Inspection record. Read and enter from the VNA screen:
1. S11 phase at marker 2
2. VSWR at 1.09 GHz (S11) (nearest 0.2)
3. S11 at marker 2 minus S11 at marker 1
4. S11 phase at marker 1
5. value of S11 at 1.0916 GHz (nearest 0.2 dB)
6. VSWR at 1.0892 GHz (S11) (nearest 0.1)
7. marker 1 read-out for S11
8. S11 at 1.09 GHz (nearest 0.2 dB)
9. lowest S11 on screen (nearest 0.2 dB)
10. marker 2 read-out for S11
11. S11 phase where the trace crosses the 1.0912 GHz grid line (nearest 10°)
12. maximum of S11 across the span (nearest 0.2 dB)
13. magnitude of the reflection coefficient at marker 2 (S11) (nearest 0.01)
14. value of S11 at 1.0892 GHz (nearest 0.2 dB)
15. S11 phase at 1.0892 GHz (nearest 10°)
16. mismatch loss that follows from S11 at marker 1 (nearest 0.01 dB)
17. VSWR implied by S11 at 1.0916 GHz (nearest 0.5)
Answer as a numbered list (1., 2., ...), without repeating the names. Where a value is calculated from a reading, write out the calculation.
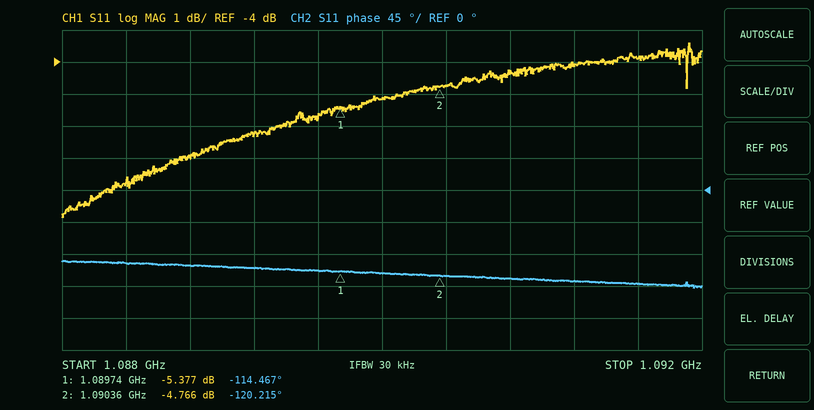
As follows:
1. -120.215°
2. |Γ| = 10^(-5.2/20) = 0.5495; VSWR = (1 + 0.5495)/(1 − 0.5495) ≈ 3.4
3. -4.766 − (-5.377) = 0.611 dB
4. -114.467°
5. -3.8 dB
6. |Γ| = 10^(-6.2/20) = 0.4898; VSWR = (1 + 0.4898)/(1 − 0.4898) ≈ 2.9
7. -5.377 dB
8. -5.2 dB
9. -8.8 dB
10. -4.766 dB
11. -130°
12. -3.4 dB
13. 10^(-4.766/20) ≈ 0.58
14. -6.2 dB
15. -110°
16. −10 log10(1 − 10^(-5.377/10)) ≈ 1.49 dB
17. |Γ| = 10^(-3.8/20) = 0.6457; VSWR = (1 + 0.6457)/(1 − 0.6457) ≈ 4.64, so 4.5 to the nearest 0.5
